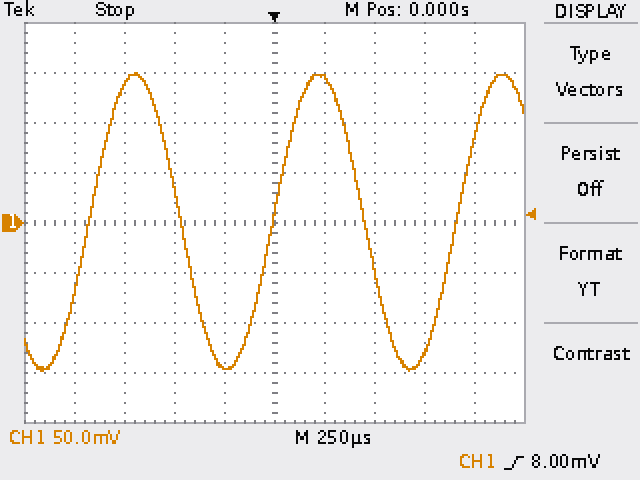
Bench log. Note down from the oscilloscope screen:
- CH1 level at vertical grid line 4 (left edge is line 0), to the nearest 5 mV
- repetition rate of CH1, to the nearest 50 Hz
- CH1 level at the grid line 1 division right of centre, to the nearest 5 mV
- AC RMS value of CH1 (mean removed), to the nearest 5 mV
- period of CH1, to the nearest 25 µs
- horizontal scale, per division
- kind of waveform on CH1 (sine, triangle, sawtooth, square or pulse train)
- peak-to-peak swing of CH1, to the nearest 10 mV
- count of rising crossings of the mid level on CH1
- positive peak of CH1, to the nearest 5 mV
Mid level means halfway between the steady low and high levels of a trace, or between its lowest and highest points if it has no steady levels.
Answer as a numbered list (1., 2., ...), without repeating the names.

1. -145 mV
2. 1.10 kHz
3. 145 mV
4. 105 mV
5. 925 µs
6. 250 µs
7. sine
8. 300 mV
9. 3
10. 150 mV
